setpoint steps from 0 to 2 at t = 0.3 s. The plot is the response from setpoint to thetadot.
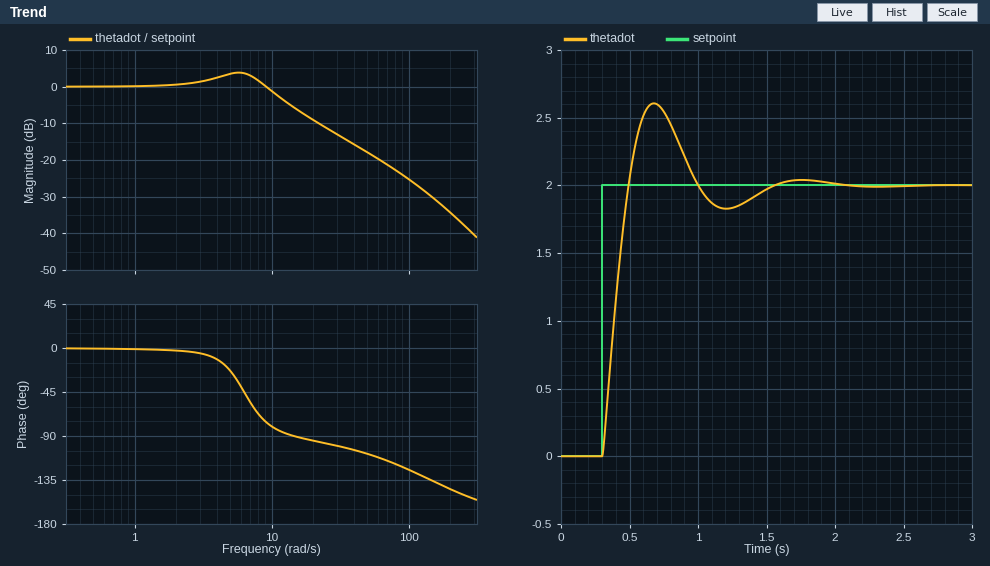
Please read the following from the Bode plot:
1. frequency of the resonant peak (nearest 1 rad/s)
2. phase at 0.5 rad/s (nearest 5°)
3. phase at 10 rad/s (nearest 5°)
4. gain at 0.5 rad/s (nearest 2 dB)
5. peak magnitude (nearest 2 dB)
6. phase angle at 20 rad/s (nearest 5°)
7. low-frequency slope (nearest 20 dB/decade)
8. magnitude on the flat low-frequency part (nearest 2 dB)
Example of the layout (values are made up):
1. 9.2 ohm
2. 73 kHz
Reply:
1. 6 rad/s
2. 0°
3. -80°
4. 0 dB
5. 4 dB
6. -95°
7. 0 dB/decade
8. 0 dB
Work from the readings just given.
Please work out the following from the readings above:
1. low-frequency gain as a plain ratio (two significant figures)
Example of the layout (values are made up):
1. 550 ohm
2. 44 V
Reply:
1. 1.0
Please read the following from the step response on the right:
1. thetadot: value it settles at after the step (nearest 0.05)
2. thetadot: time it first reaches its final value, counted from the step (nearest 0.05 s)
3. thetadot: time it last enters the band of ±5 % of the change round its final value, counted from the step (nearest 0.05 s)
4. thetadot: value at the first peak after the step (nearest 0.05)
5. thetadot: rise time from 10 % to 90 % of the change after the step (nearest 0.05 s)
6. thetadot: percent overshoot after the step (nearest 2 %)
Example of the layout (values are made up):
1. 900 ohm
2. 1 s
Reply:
1. 2.00
2. 0.20 s
3. 1.10 s
4. 2.60
5. 0.15 s
6. 30 %
